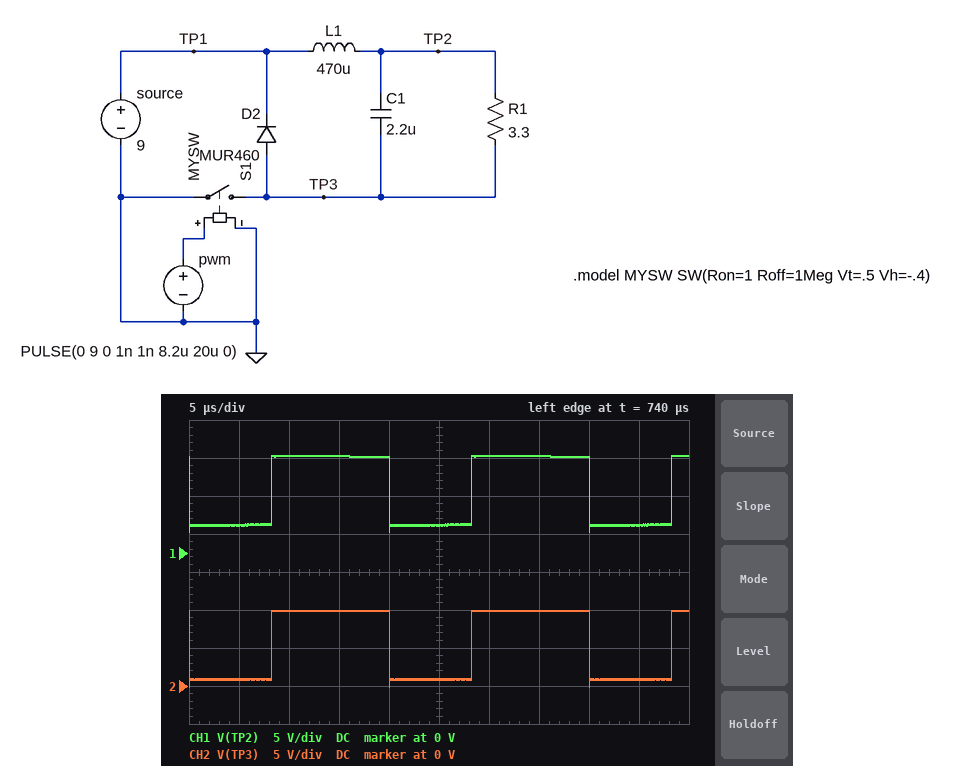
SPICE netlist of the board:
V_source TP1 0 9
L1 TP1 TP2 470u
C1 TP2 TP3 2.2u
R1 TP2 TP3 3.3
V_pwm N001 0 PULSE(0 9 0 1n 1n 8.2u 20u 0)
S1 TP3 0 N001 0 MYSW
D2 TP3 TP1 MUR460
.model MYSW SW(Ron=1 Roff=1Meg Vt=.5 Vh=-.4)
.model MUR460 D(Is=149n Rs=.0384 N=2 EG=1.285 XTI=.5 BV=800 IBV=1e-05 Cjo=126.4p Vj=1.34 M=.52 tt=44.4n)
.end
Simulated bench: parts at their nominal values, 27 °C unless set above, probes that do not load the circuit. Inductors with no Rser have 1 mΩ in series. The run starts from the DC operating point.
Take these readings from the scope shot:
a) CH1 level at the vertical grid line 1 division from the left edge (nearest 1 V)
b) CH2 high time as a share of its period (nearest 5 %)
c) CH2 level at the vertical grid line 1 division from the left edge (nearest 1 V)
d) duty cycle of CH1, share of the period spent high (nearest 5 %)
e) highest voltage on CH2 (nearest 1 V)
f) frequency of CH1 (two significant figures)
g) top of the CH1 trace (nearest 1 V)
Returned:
4 V
60 %
1 V
60 %
10 V
50 kHz
13 V
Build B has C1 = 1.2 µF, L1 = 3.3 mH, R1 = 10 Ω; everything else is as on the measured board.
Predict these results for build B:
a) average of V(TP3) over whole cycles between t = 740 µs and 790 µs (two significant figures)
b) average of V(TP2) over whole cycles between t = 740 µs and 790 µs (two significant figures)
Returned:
5.9 V
8.7 V
